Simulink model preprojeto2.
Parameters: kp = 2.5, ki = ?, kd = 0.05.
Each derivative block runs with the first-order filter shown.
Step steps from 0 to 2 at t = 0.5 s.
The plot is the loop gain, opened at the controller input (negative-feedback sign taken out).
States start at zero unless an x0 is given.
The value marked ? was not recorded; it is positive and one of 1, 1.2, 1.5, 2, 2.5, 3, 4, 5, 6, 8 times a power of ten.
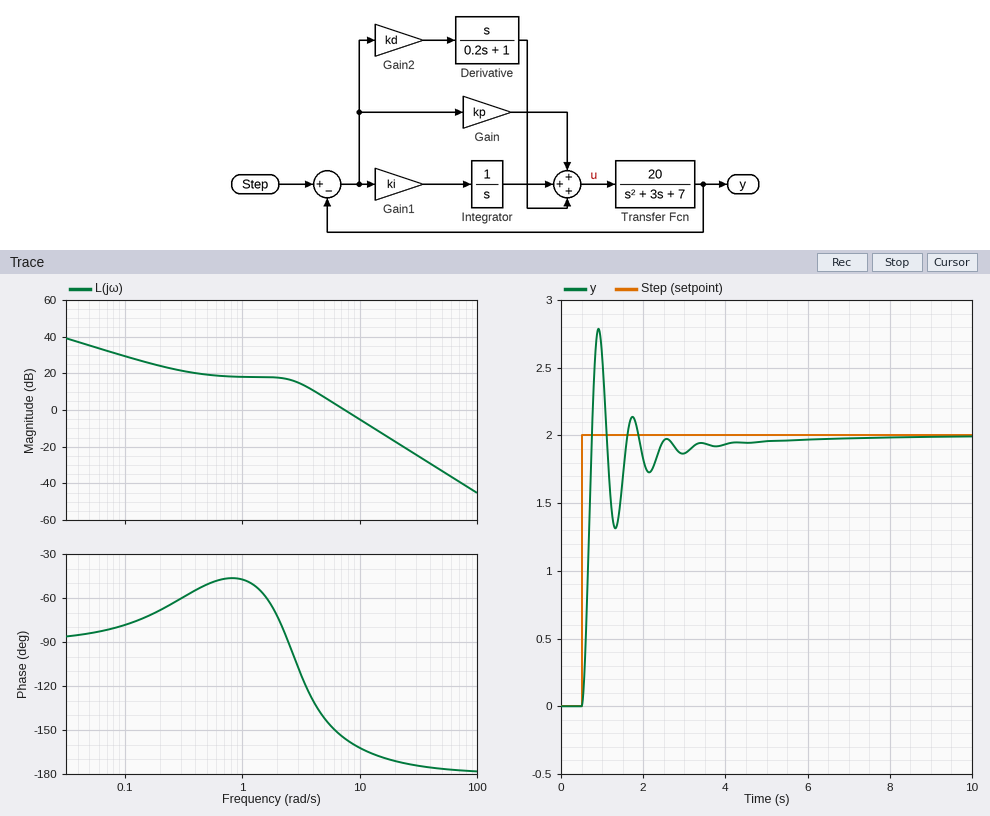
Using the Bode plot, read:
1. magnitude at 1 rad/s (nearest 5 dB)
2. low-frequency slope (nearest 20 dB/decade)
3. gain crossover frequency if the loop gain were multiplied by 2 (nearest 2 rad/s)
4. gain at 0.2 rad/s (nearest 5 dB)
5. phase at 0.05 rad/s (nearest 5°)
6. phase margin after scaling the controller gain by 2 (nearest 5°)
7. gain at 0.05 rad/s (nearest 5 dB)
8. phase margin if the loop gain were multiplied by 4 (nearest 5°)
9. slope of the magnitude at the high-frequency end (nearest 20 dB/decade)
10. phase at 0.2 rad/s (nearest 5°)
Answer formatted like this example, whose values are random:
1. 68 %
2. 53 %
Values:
1. 20 dB
2. -20 dB/decade
3. 10 rad/s
4. 25 dB
5. -85°
6. 15°
7. 35 dB
8. 10°
9. -40 dB/decade
10. -70°
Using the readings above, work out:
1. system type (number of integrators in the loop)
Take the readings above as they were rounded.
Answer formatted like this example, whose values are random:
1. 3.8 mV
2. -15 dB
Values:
1. 1
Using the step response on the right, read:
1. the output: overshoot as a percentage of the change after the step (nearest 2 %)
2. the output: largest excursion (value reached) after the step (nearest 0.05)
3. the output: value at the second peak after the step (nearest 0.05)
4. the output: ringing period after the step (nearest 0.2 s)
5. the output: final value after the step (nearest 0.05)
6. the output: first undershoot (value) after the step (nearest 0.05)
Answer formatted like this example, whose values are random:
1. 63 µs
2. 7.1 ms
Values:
1. 40 %
2. 2.80
3. 2.15
4. 0.8 s
5. 2.00
6. 1.30
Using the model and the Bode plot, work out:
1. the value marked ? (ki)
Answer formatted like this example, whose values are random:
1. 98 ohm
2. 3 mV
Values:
1. 1
